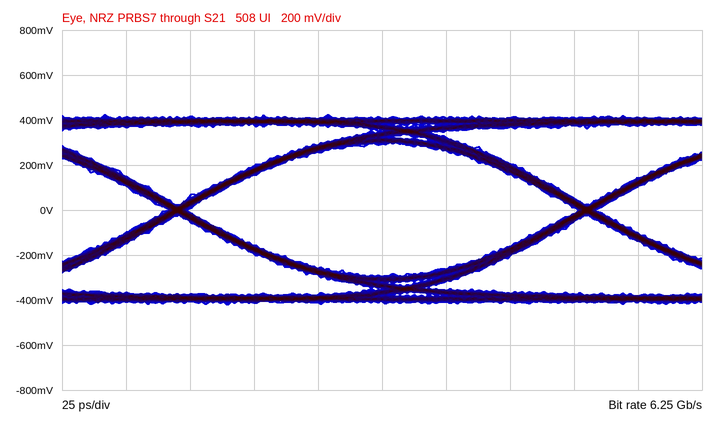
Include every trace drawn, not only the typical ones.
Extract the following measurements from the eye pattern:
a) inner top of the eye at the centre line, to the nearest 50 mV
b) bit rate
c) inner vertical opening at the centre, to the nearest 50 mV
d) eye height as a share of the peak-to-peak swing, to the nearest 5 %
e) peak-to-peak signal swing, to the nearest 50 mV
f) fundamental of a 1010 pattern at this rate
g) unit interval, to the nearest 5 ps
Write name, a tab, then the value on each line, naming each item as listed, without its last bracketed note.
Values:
inner top of the eye at the centre line, to the nearest 50 mV	300 mV
bit rate	6.25 Gb/s
inner vertical opening at the centre, to the nearest 50 mV	600 mV
eye height as a share of the peak-to-peak swing, to the nearest 5 %	70 %
peak-to-peak signal swing, to the nearest 50 mV	850 mV
fundamental of a 1010 pattern at this rate	3.125 GHz
unit interval, to the nearest 5 ps	160 ps
